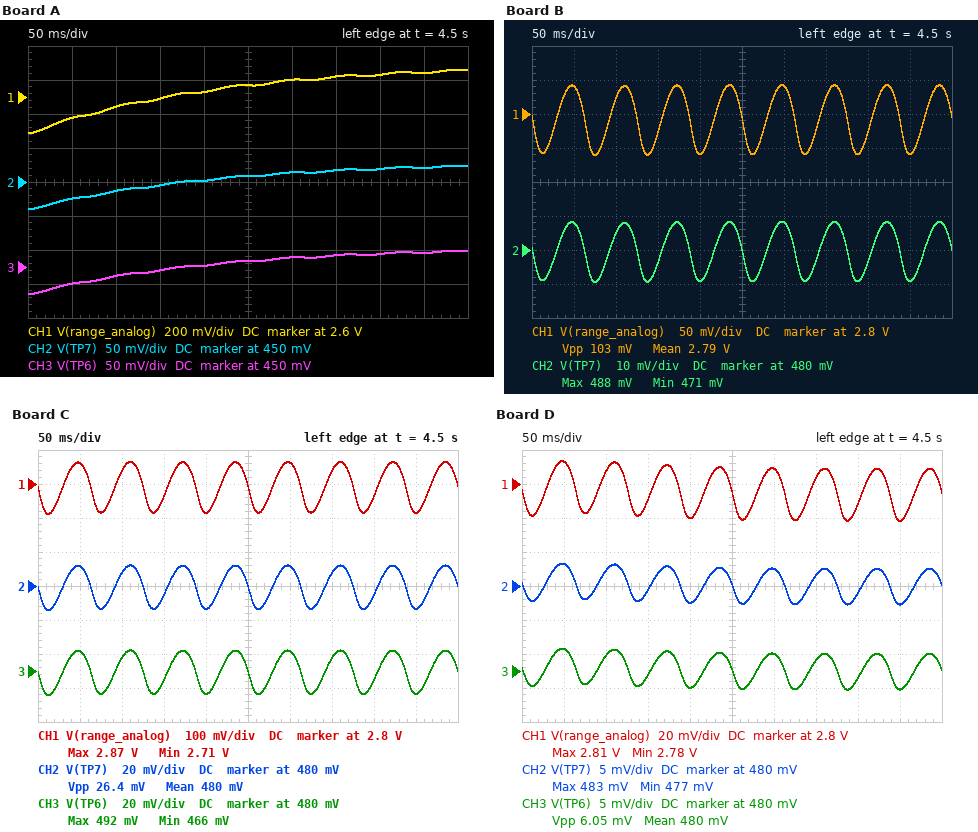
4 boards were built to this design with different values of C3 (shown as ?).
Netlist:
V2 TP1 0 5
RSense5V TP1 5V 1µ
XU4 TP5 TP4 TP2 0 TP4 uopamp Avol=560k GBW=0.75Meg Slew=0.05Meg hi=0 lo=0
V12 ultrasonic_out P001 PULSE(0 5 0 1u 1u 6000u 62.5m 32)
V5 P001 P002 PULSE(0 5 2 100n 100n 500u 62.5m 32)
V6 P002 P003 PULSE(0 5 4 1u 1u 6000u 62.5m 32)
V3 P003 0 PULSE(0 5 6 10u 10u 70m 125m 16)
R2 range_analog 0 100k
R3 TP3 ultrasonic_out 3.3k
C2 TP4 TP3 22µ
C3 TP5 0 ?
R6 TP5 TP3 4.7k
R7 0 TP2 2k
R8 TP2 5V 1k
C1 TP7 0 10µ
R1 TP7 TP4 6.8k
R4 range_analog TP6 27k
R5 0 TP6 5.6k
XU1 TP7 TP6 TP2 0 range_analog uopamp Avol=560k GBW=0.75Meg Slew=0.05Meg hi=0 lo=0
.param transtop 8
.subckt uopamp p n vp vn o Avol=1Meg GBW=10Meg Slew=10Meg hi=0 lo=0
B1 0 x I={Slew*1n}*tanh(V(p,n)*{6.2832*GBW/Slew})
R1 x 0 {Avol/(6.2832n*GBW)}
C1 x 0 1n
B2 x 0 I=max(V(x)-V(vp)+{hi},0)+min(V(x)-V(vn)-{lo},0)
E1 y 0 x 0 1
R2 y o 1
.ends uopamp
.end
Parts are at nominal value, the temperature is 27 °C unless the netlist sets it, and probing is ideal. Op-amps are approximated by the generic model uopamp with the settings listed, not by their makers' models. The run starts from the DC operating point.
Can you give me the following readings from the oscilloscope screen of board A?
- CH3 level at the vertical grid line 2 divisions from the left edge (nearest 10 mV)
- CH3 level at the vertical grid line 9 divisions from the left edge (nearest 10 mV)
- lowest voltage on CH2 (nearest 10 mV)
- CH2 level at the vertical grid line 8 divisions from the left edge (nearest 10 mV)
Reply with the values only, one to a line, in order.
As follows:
440 mV
470 mV
410 mV
470 mV
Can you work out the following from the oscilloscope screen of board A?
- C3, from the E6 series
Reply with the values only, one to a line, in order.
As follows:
33 µF
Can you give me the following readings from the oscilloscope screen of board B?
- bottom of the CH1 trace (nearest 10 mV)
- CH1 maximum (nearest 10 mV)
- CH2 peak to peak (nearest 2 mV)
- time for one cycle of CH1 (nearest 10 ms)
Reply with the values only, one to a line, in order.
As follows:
2.74 V
2.84 V
18 mV
60 ms
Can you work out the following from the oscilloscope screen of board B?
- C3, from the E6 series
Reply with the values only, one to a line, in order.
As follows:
4.7 µF
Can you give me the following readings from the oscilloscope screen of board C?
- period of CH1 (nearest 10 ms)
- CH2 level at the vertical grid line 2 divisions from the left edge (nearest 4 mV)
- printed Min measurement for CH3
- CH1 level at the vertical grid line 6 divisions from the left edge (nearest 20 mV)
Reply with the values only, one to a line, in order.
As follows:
60 ms
488 mV
466 mV
2.86 V
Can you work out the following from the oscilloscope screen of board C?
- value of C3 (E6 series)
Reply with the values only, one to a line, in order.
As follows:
3.3 µF
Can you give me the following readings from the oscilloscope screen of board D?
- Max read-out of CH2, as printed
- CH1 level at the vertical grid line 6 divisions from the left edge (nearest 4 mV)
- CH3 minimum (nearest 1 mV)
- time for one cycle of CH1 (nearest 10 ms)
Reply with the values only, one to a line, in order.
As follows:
483 mV
2.808 V
477 mV
60 ms
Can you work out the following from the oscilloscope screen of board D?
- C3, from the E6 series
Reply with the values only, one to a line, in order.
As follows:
15 µF
